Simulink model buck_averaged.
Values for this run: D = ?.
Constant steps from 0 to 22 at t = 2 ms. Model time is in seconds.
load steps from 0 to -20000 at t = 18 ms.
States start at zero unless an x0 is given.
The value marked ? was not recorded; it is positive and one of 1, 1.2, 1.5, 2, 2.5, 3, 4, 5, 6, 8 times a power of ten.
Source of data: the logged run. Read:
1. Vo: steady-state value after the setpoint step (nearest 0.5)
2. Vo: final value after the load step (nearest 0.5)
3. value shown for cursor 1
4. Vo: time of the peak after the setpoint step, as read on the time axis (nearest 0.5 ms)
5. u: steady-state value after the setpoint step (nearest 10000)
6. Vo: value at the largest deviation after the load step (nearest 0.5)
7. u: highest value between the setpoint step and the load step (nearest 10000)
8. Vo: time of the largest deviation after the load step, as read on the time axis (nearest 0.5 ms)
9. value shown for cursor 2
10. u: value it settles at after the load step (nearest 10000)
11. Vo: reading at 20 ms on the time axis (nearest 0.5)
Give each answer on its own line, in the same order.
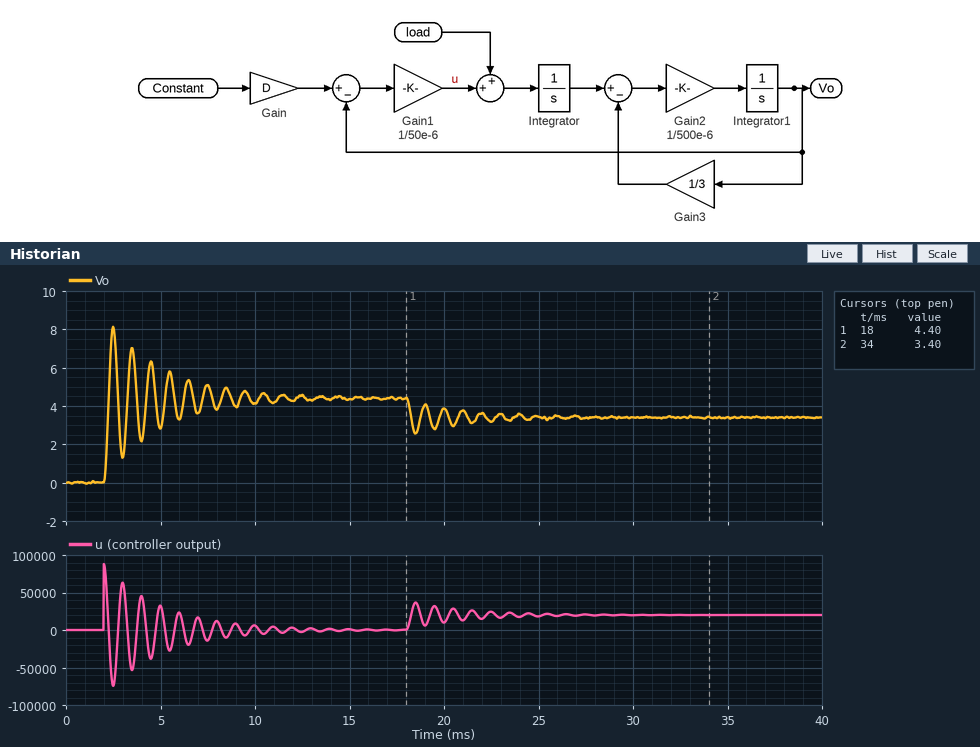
4.5
3.5
4.40
2.5 ms
0
2.5
90000
18.5 ms
3.40
20000
4.0
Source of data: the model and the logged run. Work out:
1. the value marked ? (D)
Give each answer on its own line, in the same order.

0.2
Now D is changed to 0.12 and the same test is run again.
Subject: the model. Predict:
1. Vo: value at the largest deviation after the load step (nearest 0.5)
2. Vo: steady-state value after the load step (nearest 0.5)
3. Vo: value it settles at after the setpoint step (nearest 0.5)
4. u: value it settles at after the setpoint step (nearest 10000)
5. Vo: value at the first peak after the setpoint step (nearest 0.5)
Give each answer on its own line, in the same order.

1.0
1.5
2.5
0
5.0
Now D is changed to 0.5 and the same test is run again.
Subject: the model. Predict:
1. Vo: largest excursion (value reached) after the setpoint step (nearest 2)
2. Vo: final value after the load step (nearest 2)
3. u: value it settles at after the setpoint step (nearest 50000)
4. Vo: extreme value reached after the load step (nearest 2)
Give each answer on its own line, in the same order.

20
10
0
10
